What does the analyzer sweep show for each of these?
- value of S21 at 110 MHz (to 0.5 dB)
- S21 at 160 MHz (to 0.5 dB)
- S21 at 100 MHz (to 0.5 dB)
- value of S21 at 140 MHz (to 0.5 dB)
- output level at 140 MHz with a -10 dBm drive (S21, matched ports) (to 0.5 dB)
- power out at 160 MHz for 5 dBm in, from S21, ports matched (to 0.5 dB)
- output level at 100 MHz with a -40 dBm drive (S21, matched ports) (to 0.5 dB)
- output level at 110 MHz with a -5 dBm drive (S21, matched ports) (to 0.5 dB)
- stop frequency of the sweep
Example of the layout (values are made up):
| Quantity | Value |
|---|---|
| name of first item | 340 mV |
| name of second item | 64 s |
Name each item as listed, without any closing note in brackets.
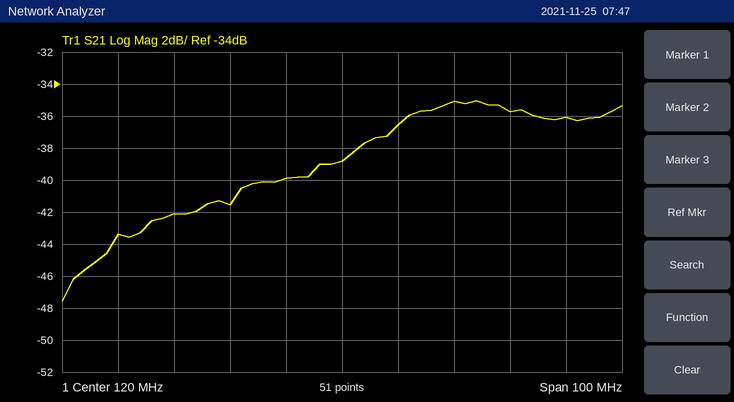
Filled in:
| Quantity | Value |
|---|---|
| value of S21 at 110 MHz | -40.0 dB |
| S21 at 160 MHz | -36.0 dB |
| S21 at 100 MHz | -41.5 dB |
| value of S21 at 140 MHz | -35.0 dB |
| output level at 140 MHz with a -10 dBm drive (S21, matched ports) | -45.0 dBm |
| power out at 160 MHz for 5 dBm in, from S21, ports matched | -31.0 dBm |
| output level at 100 MHz with a -40 dBm drive (S21, matched ports) | -81.5 dBm |
| output level at 110 MHz with a -5 dBm drive (S21, matched ports) | -45.0 dBm |
| stop frequency of the sweep | 170 MHz |
